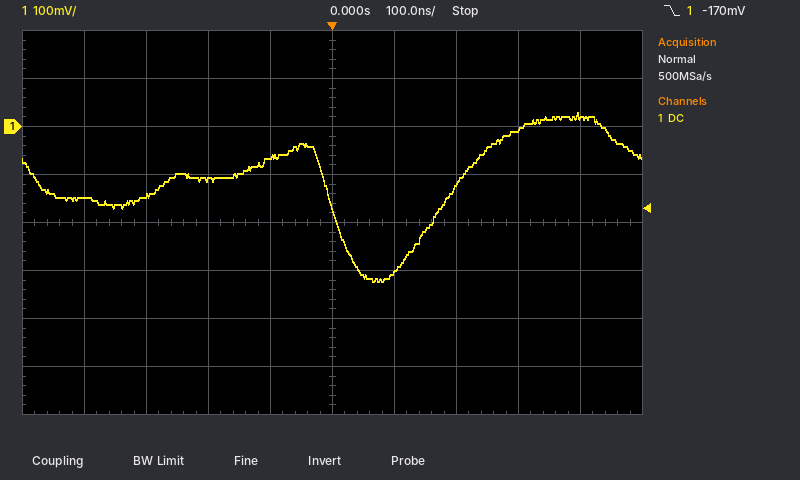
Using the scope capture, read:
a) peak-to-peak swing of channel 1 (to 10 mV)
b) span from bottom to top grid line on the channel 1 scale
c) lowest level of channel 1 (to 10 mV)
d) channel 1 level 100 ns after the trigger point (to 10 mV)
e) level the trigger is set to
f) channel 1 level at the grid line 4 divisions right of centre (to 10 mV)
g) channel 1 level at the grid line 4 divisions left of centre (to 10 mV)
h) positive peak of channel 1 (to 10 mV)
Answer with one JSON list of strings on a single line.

["350 mV", "800 mV", "-320 mV", "-300 mV", "-170 mV", "20 mV", "-150 mV", "30 mV"]
